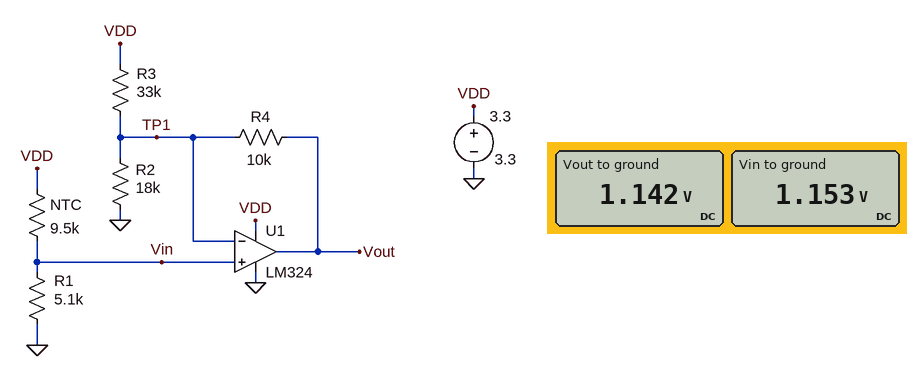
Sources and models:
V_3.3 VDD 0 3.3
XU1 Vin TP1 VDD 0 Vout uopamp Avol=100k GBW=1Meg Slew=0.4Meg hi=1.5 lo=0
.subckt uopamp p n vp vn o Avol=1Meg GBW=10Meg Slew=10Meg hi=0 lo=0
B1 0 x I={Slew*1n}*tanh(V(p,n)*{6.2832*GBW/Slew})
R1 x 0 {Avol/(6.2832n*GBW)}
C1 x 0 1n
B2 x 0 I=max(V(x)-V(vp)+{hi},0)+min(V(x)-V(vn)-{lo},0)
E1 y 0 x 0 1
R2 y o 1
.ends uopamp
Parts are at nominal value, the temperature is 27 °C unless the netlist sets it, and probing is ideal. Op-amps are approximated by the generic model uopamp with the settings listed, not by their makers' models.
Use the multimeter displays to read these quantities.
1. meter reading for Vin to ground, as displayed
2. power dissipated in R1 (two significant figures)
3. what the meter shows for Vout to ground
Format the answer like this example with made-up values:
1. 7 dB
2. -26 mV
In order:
1. 1.153 V
2. 260 µW
3. 1.142 V
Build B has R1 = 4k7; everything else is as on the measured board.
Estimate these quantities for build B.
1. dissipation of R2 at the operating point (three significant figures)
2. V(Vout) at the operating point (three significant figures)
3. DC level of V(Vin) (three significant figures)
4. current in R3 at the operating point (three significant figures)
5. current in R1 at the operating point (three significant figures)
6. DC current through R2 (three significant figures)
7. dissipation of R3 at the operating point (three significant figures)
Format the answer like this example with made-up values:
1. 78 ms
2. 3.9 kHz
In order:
1. 66.3 µW
2. 1.03 V
3. 1.09 V
4. 66.9 µA
5. 232 µA
6. 60.7 µA
7. 148 µW
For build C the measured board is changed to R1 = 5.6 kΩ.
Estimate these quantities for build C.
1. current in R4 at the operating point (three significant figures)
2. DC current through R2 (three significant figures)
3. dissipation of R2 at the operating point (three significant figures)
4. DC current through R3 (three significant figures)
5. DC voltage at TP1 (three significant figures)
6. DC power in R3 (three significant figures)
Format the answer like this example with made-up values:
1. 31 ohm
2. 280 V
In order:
1. 5.08 µA
2. 68.0 µA
3. 83.2 µW
4. 62.9 µA
5. 1.22 V
6. 131 µW
